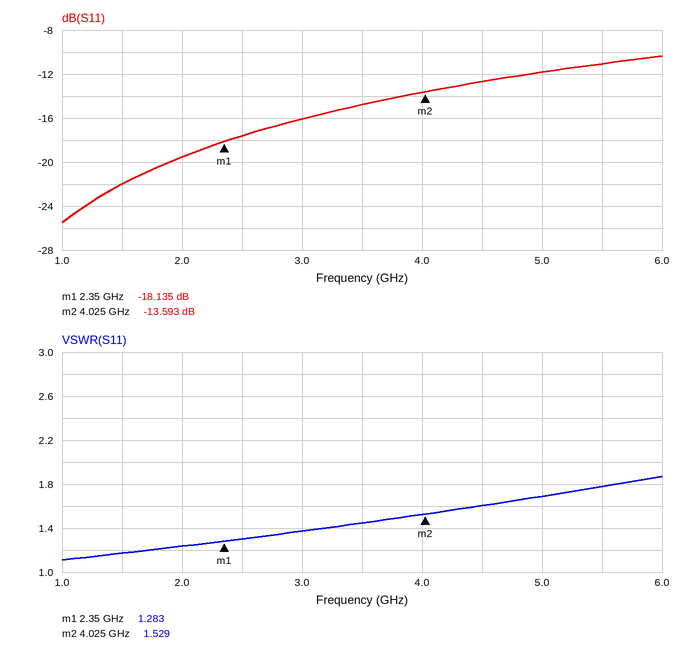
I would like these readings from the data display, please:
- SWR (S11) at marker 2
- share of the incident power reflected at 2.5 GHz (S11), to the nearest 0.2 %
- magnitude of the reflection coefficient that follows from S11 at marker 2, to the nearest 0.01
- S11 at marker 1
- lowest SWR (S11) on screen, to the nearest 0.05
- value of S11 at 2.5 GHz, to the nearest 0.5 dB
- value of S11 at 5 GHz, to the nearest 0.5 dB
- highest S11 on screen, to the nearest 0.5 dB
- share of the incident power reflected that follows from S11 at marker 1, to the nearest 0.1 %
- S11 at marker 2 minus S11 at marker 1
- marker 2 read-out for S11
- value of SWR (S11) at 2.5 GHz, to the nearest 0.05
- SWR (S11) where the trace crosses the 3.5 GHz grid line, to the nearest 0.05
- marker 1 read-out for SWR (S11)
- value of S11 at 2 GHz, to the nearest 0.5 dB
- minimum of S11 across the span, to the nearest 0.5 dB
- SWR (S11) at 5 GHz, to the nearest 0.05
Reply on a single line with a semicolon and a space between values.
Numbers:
1.529; 1.8 %; 0.21; -18.135 dB; 1.10; -17.5 dB; -12.0 dB; -10.5 dB; 1.5 %; 4.542 dB; -13.593 dB; 1.30; 1.45; 1.283; -19.5 dB; -25.5 dB; 1.70
